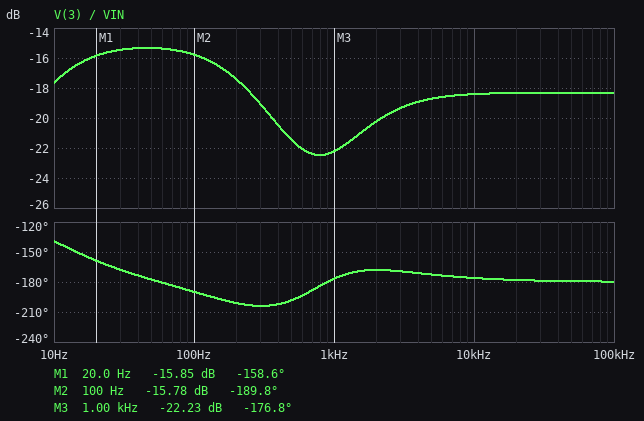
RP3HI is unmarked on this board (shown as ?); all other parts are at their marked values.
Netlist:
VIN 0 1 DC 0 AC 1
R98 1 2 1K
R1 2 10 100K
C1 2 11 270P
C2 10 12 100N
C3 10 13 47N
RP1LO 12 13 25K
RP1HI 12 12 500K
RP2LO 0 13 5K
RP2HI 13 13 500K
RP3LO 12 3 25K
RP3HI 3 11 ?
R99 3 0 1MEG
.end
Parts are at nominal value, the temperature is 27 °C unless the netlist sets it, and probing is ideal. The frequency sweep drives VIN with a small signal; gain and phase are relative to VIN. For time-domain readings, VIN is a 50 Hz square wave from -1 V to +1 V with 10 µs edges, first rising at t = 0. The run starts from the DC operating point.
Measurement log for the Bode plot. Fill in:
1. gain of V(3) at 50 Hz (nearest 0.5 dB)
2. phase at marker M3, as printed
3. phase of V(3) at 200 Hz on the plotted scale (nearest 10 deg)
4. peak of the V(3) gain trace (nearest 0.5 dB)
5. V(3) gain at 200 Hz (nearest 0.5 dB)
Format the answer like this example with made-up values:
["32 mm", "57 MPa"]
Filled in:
["-15.5 dB", "-176.8 deg", "-200 deg", "-15.5 dB", "-17.5 dB"]
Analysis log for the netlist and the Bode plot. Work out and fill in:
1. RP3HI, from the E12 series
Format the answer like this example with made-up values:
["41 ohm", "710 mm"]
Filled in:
["330 kΩ"]
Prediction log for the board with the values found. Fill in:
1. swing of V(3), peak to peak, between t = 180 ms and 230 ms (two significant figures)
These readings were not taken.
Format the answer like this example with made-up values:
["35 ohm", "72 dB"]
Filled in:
["390 mV"]
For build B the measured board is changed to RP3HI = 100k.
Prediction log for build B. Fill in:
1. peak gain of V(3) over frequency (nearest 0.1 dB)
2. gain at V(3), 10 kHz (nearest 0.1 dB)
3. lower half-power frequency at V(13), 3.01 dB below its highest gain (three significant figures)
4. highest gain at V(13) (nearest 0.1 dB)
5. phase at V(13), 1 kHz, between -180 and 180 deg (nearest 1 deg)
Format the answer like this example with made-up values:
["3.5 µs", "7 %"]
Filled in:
["-11.8 dB", "-12.7 dB", "2.61 kHz", "-21.9 dB", "-170 deg"]
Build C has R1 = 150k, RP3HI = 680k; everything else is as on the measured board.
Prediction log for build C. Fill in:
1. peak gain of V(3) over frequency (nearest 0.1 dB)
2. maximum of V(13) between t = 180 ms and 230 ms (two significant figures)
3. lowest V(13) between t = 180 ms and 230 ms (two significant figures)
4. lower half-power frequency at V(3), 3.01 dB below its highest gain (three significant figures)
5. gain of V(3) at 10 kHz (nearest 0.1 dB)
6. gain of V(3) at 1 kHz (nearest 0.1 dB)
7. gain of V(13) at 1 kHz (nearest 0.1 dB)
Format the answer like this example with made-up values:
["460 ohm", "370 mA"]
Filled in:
["-18.3 dB", "53 mV", "-53 mV", "6.12 Hz", "-23.1 dB", "-24.2 dB", "-29.0 dB"]
